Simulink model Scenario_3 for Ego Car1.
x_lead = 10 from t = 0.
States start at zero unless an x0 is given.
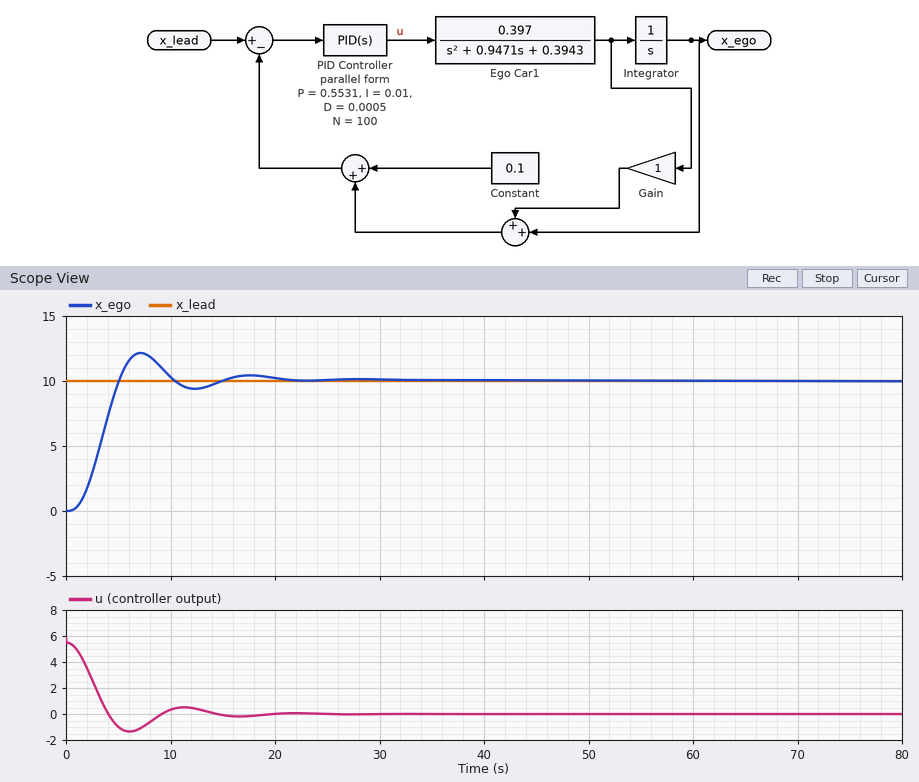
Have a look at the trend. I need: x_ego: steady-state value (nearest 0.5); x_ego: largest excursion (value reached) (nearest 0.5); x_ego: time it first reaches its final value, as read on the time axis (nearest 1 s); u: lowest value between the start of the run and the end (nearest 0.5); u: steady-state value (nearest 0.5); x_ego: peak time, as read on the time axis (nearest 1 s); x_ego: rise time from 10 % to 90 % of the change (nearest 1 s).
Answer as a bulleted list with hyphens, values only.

- 10.0
- 12.0
- 5 s
- -1.5
- 0.0
- 7 s
- 3 s
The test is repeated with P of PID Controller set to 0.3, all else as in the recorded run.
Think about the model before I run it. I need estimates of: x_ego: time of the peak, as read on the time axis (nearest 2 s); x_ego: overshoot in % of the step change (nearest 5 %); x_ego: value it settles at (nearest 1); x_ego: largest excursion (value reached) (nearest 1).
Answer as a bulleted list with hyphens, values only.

- 10 s
- 15 %
- 10
- 11
